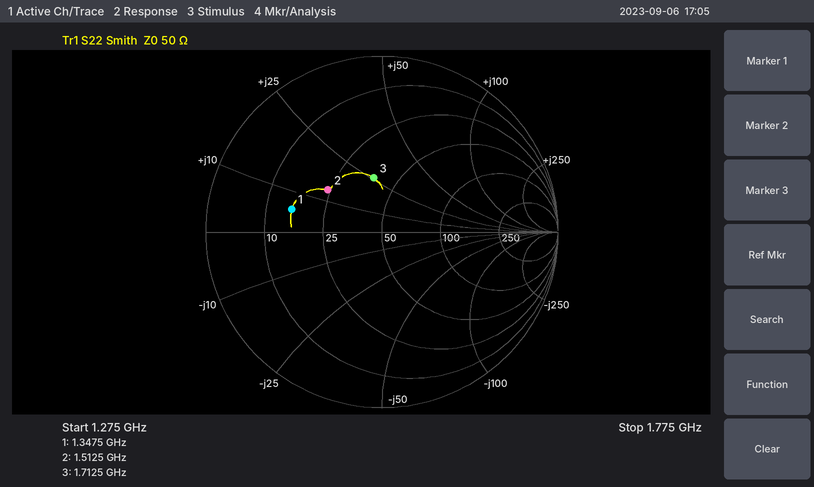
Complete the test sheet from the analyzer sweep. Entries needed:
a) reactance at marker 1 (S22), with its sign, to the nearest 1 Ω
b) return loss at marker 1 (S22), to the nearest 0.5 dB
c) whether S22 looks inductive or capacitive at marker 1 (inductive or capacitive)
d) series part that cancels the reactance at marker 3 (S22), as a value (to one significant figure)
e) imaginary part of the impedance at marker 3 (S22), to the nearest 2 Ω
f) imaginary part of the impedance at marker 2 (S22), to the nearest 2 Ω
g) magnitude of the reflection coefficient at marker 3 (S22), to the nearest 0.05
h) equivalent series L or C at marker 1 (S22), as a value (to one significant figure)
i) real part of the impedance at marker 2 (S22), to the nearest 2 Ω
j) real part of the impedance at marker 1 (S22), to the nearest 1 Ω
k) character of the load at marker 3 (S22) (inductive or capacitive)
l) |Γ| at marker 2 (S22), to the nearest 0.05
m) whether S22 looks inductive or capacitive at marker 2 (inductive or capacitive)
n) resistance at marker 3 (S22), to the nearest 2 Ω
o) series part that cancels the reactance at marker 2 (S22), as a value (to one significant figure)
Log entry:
+6 Ω
5.5 dB
inductive
4 pF
+26 Ω
+14 Ω
0.30
700 pH
24 Ω
16 Ω
inductive
0.40
inductive
38 Ω
8 pF
